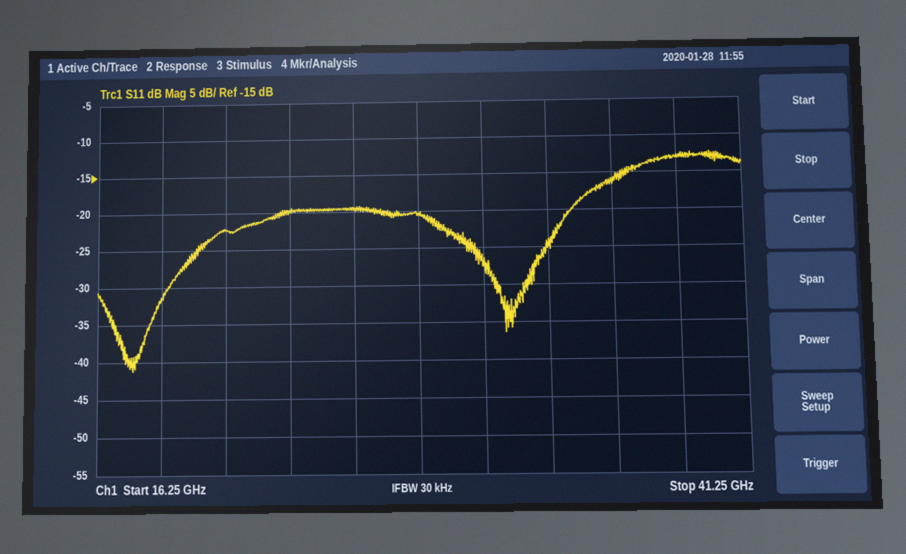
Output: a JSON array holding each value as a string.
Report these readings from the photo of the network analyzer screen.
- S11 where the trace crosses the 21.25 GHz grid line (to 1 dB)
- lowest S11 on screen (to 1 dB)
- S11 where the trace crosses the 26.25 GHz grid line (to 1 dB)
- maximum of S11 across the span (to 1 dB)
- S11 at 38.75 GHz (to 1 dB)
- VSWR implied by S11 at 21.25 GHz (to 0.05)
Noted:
["-22 dB", "-41 dB", "-20 dB", "-12 dB", "-13 dB", "1.15"]
